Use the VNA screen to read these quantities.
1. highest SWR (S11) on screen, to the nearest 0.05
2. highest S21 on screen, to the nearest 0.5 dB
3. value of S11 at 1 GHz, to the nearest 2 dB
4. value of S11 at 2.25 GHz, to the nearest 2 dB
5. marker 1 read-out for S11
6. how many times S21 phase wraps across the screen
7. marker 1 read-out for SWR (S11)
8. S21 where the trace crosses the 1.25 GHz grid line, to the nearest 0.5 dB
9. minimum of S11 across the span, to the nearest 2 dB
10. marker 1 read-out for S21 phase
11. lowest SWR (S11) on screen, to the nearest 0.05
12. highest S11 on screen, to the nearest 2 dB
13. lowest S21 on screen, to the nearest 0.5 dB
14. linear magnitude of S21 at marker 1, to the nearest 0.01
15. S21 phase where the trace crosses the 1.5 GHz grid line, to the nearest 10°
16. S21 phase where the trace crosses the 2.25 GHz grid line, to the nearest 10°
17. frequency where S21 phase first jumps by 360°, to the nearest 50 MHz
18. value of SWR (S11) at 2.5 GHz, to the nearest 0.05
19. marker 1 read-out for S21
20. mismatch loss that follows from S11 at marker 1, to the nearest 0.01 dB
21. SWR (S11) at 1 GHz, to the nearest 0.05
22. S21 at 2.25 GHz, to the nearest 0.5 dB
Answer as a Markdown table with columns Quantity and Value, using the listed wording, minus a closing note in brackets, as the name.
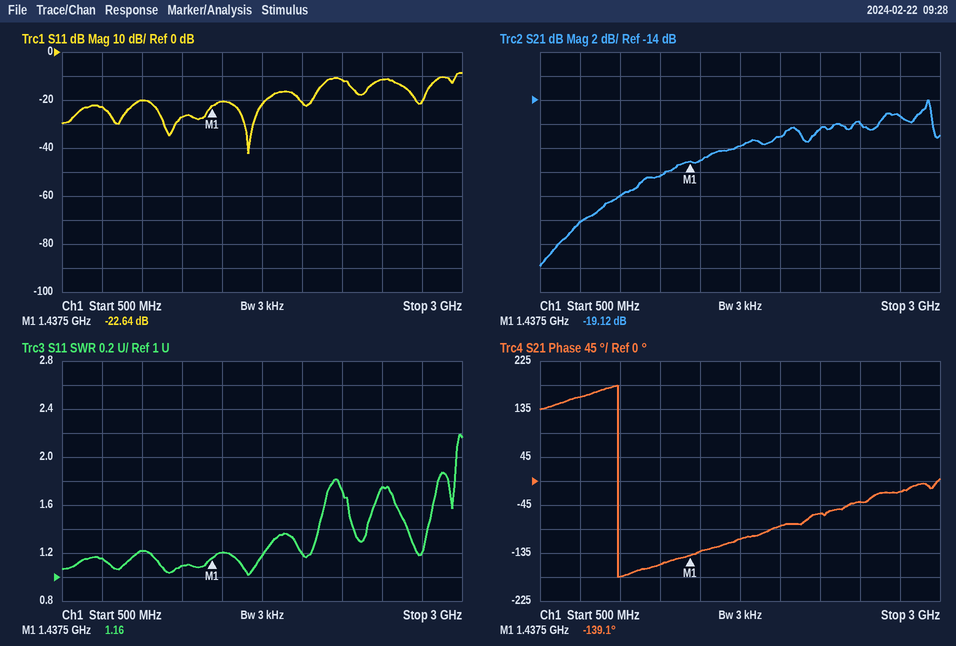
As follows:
| Quantity | Value |
|---|---|
| highest SWR (S11) on screen, to the nearest 0.05 | 2.20 |
| highest S21 on screen, to the nearest 0.5 dB | -14.0 dB |
| value of S11 at 1 GHz, to the nearest 2 dB | -20 dB |
| value of S11 at 2.25 GHz, to the nearest 2 dB | -12 dB |
| marker 1 read-out for S11 | -22.64 dB |
| how many times S21 phase wraps across the screen | 1 |
| marker 1 read-out for SWR | 1.16 |
| S21 where the trace crosses the 1.25 GHz grid line, to the nearest 0.5 dB | -20.5 dB |
| minimum of S11 across the span, to the nearest 2 dB | -42 dB |
| marker 1 read-out for S21 phase | -139.1° |
| lowest SWR (S11) on screen, to the nearest 0.05 | 1.00 |
| highest S11 on screen, to the nearest 2 dB | -8 dB |
| lowest S21 on screen, to the nearest 0.5 dB | -28.0 dB |
| linear magnitude of S21 at marker 1, to the nearest 0.01 | 0.11 |
| S21 phase where the trace crosses the 1.5 GHz grid line, to the nearest 10° | -130° |
| S21 phase where the trace crosses the 2.25 GHz grid line, to the nearest 10° | -60° |
| frequency where S21 phase first jumps by 360°, to the nearest 50 MHz | 1.00 GHz |
| value of SWR (S11) at 2.5 GHz, to the nearest 0.05 | 1.75 |
| marker 1 read-out for S21 | -19.12 dB |
| mismatch loss that follows from S11 at marker 1, to the nearest 0.01 dB | 0.02 dB |
| SWR (S11) at 1 GHz, to the nearest 0.05 | 1.20 |
| S21 at 2.25 GHz, to the nearest 0.5 dB | -16.5 dB |
